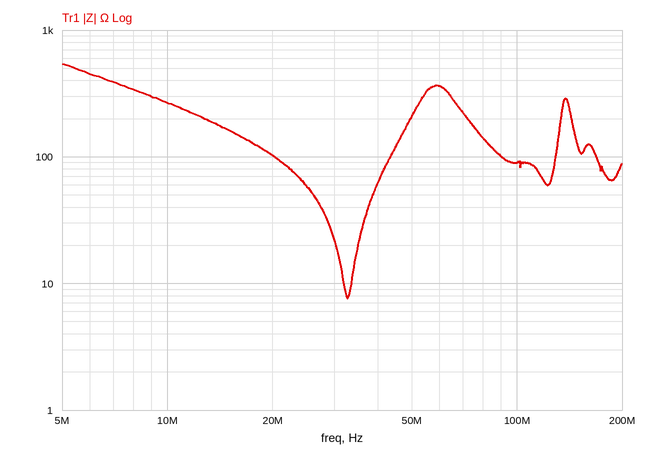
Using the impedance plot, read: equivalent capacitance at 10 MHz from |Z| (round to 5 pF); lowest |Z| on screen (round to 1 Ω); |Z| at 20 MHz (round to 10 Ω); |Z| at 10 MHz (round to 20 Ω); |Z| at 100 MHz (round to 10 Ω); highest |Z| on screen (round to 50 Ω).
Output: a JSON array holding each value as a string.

["60 pF", "8 Ω", "100 Ω", "260 Ω", "90 Ω", "550 Ω"]
